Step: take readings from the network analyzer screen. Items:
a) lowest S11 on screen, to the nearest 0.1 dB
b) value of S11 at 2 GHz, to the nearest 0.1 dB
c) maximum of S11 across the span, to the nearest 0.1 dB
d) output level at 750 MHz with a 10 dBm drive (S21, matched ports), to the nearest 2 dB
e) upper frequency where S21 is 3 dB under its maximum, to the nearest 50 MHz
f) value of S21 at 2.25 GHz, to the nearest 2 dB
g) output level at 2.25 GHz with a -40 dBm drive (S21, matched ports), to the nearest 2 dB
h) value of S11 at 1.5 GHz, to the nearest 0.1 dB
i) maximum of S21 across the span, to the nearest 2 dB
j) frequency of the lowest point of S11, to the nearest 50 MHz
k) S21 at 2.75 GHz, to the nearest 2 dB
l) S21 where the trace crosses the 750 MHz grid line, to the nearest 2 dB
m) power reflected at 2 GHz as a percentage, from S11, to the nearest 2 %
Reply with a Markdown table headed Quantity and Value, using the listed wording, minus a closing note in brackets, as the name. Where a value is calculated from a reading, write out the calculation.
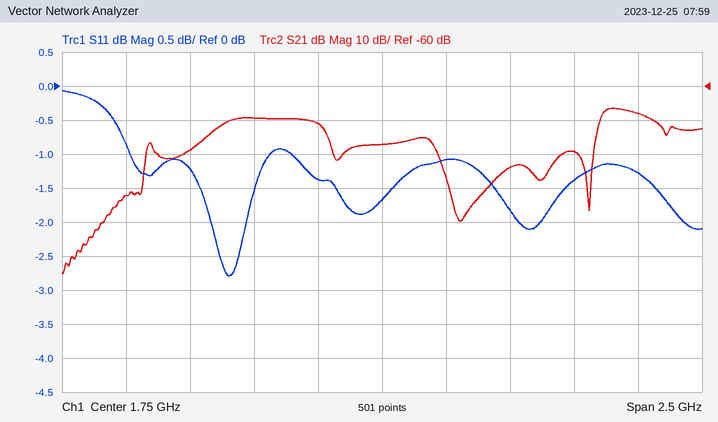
| Quantity | Value |
|---|---|
| lowest S11 on screen, to the nearest 0.1 dB | -2.8 dB |
| value of S11 at 2 GHz, to the nearest 0.1 dB | -1.1 dB |
| maximum of S11 across the span, to the nearest 0.1 dB | -0.1 dB |
| output level at 750 MHz with a 10 dBm drive (S21, matched ports), to the nearest 2 dB | 10 dBm + (-92 dB) = -82 dBm |
| upper frequency where S21 is 3 dB under its maximum, to the nearest 50 MHz | 2.80 GHz |
| value of S21 at 2.25 GHz, to the nearest 2 dB | -84 dB |
| output level at 2.25 GHz with a -40 dBm drive (S21, matched ports), to the nearest 2 dB | -40 dBm + (-84 dB) = -124 dBm |
| value of S11 at 1.5 GHz, to the nearest 0.1 dB | -1.4 dB |
| maximum of S21 across the span, to the nearest 2 dB | -66 dB |
| frequency of the lowest point of S11, to the nearest 50 MHz | 1.15 GHz |
| S21 at 2.75 GHz, to the nearest 2 dB | -68 dB |
| S21 where the trace crosses the 750 MHz grid line, to the nearest 2 dB | -92 dB |
| power reflected at 2 GHz as a percentage, from S11, to the nearest 2 % | 10^(-1.1/10) ≈ 78 % |
